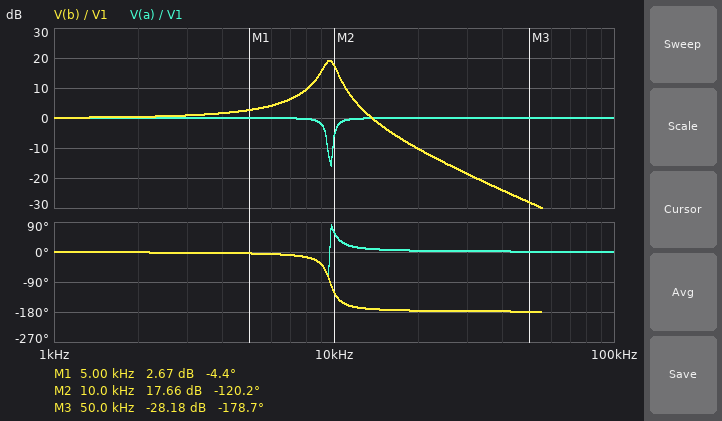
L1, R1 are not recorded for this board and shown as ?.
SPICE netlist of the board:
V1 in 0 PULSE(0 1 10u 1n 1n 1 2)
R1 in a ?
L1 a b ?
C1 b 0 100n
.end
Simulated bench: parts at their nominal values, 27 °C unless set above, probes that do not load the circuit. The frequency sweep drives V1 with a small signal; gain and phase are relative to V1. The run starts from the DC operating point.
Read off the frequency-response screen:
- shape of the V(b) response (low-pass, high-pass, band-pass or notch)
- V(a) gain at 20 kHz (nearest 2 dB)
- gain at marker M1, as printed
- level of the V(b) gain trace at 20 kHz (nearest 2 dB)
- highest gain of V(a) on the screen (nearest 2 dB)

low-pass
0 dB
2.67 dB
-10 dB
0 dB
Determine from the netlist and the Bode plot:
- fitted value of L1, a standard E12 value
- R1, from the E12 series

2.7 mH
18 Ω
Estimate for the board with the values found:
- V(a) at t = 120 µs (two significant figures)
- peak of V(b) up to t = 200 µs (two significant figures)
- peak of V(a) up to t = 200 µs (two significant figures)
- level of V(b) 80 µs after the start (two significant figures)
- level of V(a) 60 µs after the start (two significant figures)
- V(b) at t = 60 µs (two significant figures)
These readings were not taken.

970 mV
1.8 V
1.1 V
1.4 V
990 mV
1.8 V
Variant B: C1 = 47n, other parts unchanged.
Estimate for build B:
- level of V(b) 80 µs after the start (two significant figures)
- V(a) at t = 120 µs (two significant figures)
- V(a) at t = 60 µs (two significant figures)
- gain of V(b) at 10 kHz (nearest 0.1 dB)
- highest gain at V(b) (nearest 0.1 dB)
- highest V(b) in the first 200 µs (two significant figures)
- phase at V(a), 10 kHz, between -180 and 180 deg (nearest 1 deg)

210 mV
1.0 V
1.1 V
6.0 dB
22.5 dB
1.9 V
-6 deg
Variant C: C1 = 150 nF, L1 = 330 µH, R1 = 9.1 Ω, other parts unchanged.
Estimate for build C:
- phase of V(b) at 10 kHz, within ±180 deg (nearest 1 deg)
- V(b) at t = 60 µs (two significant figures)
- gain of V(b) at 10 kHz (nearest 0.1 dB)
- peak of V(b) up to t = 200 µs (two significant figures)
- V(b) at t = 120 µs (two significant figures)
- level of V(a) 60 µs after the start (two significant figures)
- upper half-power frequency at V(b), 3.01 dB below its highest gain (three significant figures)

-6 deg
610 mV
1.8 dB
1.7 V
1.2 V
930 mV
24.5 kHz
